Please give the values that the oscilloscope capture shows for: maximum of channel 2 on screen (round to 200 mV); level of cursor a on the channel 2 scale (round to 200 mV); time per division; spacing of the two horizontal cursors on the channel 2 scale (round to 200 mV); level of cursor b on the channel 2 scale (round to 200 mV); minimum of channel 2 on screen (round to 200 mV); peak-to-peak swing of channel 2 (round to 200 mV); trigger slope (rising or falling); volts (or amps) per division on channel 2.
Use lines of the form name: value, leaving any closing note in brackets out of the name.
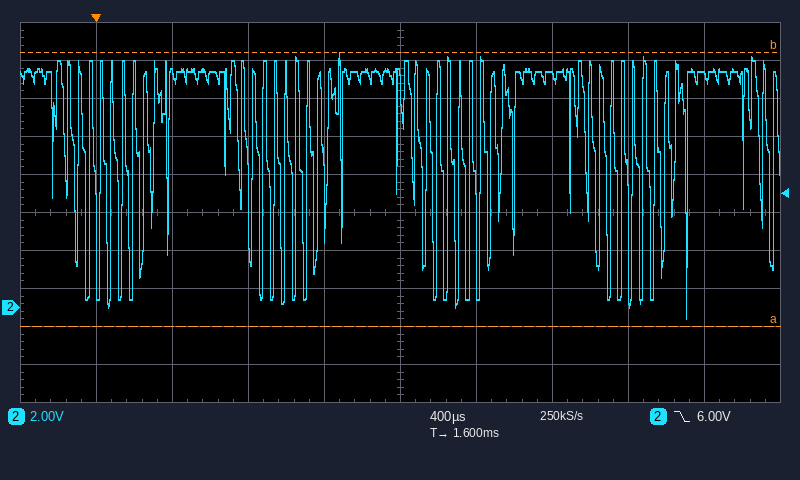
maximum of channel 2 on screen: 13.4 V
level of cursor a on the channel 2 scale: -1.0 V
time per division: 400 µs
spacing of the two horizontal cursors on the channel 2 scale: 14.4 V
level of cursor b on the channel 2 scale: 13.4 V
minimum of channel 2 on screen: -600 mV
peak-to-peak swing of channel 2: 14.0 V
trigger slope: falling
volts (or amps) per division on channel 2: 2 V
